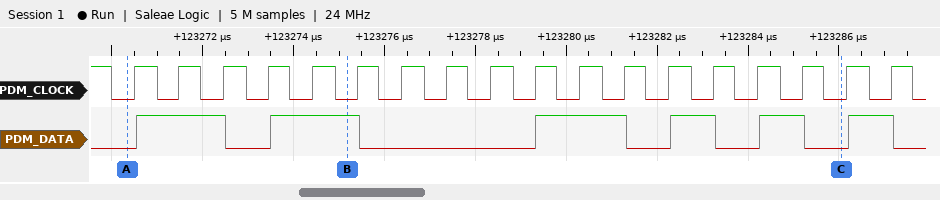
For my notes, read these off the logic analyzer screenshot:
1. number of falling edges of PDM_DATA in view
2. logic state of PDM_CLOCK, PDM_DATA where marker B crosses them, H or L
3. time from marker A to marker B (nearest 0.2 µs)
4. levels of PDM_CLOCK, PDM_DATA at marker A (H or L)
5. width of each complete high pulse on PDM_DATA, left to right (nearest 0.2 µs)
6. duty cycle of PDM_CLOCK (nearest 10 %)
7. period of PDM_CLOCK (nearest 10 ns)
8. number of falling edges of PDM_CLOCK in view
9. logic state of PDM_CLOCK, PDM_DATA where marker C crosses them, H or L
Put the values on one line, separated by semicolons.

6; PDM_CLOCK=L, PDM_DATA=H; 4.8 µs; PDM_CLOCK=L, PDM_DATA=L; 2 µs, 2 µs, 2 µs, 1 µs, 1 µs, 1 µs; 50 %; 980 ns; 19; PDM_CLOCK=L, PDM_DATA=L
